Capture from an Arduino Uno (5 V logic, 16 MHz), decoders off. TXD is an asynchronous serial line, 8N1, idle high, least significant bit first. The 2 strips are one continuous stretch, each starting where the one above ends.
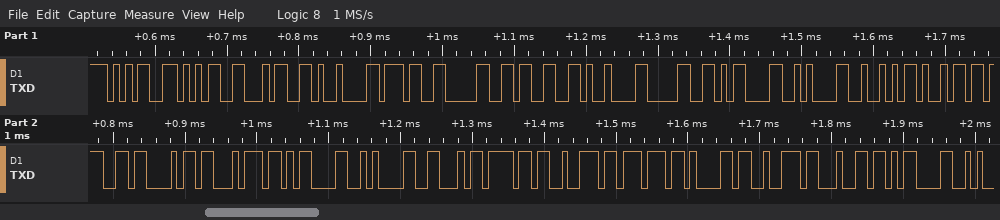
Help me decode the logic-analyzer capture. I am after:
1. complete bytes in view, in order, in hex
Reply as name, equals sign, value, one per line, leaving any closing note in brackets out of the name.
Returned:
complete bytes in view, in order, in hex = 0x35 0x35 0x34 0x09 0x37 0x30 0x33 0x09 0x30 0x0D 0x0A 0x52 0x69 0x67 0x68 0x74 0x0D 0x0A 0x46 0x6F 0x72 0x77 0x61 0x72 0x64 0x0D
